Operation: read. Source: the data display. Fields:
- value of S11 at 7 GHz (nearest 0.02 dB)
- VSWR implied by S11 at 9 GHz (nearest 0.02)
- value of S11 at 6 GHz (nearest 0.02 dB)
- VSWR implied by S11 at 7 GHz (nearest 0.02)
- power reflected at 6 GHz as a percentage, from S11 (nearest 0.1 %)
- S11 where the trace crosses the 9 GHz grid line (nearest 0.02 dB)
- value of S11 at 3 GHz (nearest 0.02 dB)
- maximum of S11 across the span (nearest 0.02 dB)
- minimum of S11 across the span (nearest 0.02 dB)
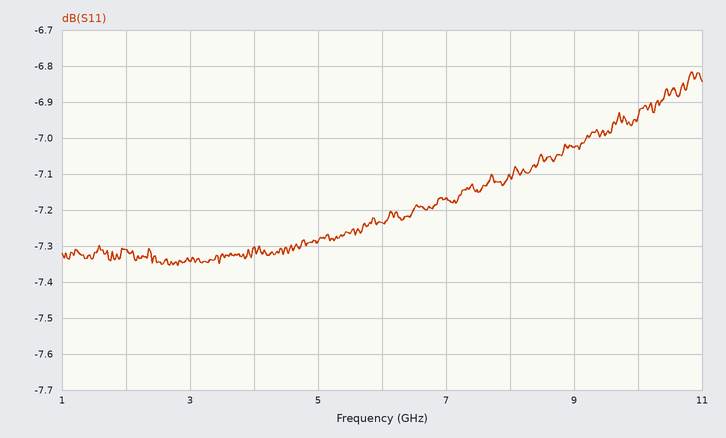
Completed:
-7.16 dB
2.60
-7.24 dB
2.56
18.9 %
-7.02 dB
-7.34 dB
-6.82 dB
-7.36 dB
